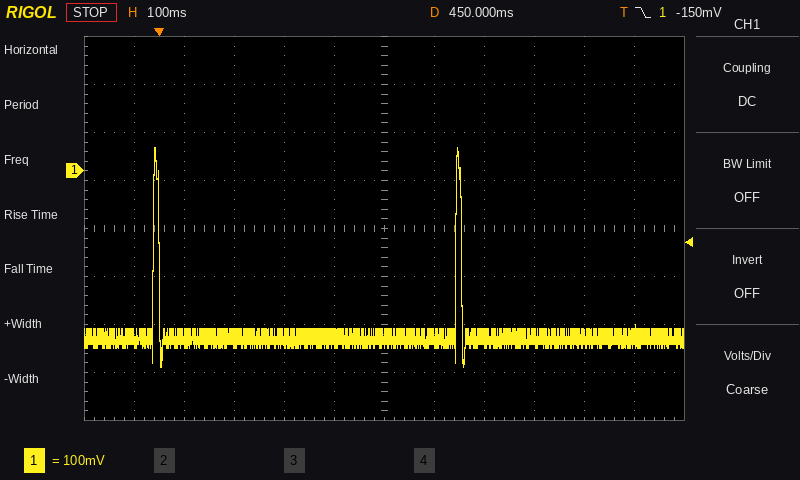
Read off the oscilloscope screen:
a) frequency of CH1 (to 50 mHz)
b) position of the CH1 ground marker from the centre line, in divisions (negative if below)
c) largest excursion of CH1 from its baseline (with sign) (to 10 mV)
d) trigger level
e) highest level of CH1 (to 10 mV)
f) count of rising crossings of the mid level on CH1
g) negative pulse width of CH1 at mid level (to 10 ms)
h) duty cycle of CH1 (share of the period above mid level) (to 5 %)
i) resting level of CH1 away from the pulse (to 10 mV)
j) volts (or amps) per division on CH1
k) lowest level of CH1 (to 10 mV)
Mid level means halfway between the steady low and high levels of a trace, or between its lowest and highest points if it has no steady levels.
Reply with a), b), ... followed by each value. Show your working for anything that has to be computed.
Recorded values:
a) 1.65 Hz
b) +1.2 div
c) 50 mV − (-350 mV) = +400 mV
d) -150 mV
e) 50 mV
f) 2
g) 590 ms
h) 0 %
i) -350 mV
j) 100 mV
k) -410 mV
